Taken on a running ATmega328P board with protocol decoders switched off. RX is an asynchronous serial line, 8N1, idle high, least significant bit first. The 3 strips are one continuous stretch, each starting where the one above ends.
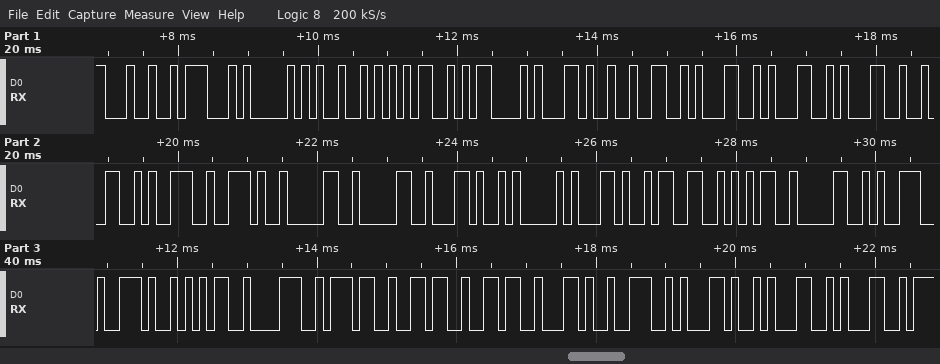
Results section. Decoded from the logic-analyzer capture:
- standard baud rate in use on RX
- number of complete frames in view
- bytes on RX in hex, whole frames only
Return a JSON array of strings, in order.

["9600 baud", "34", "24 47 50 52 4D 43 2C 32 31 31 31 32 39 2E 30 30 2C 41 2C 33 35 30 39 2E 35 38 37 36 36 2C 4E 2C 31 31"]
